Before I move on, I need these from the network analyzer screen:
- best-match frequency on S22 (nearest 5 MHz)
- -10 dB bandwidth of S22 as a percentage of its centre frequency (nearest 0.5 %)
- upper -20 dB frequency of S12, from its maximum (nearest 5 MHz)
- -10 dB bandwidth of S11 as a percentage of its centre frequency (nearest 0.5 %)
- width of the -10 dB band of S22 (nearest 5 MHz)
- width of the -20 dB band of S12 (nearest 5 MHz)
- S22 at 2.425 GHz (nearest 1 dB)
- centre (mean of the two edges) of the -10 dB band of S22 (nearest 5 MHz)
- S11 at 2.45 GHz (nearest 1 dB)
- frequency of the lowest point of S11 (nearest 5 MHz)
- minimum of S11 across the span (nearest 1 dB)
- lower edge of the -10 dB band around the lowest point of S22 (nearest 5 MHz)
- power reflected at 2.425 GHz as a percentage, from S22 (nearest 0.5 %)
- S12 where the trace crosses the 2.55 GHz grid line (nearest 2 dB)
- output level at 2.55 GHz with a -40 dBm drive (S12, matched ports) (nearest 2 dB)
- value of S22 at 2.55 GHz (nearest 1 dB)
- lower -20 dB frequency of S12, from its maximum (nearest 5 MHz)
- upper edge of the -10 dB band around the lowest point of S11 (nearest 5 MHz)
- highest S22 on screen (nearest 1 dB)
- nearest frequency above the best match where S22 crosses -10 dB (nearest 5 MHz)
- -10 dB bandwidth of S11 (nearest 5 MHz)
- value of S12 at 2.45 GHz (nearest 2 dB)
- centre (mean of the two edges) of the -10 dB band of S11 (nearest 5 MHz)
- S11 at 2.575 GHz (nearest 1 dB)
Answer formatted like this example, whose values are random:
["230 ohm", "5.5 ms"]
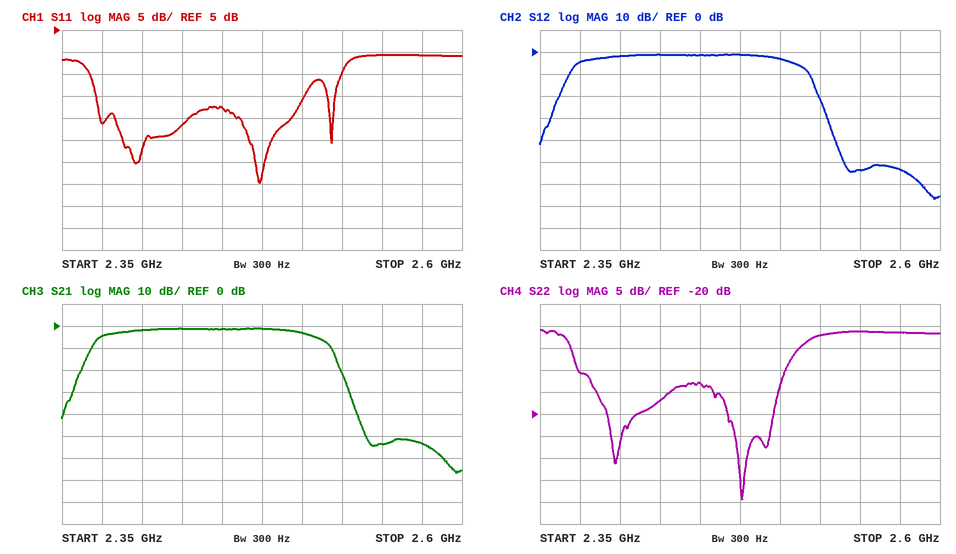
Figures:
["2.475 GHz", "5.5 %", "2.525 GHz", "5.5 %", "130 MHz", "165 MHz", "-17 dB", "2.440 GHz", "-13 dB", "2.475 GHz", "-30 dB", "2.375 GHz", "2.0 %", "-54 dB", "-94 dBm", "-1 dB", "2.360 GHz", "2.500 GHz", "-1 dB", "2.505 GHz", "130 MHz", "-2 dB", "2.435 GHz", "-1 dB"]
